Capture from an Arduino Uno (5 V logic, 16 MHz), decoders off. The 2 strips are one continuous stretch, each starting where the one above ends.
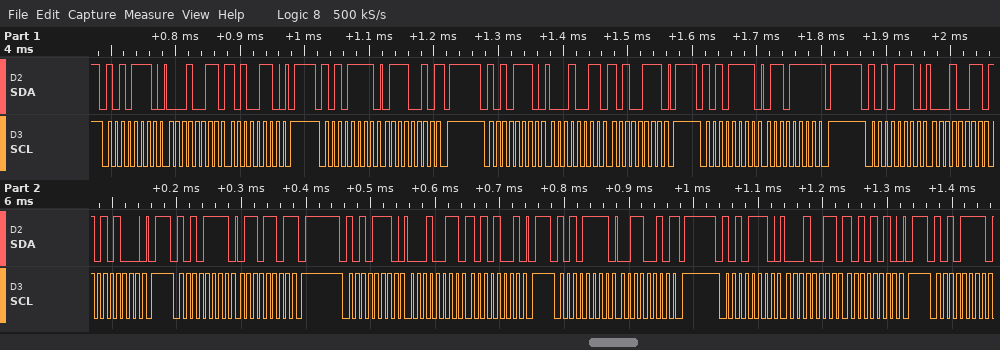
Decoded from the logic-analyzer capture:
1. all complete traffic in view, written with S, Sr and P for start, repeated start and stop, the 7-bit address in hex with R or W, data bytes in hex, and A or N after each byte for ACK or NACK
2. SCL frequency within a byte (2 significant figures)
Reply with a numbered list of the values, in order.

1. S 57W A 13 A A6 A P S 57R A 72 N P S 57W A 13 A A7 A P S 57R A 6F N P S 57W A 13 A A8 A P S 57R A 6D N P S 57W A 13 A A9 A P S 57R A 32 N P S 57W A 13 A AA A P S 57R A
2. 100 kHz
